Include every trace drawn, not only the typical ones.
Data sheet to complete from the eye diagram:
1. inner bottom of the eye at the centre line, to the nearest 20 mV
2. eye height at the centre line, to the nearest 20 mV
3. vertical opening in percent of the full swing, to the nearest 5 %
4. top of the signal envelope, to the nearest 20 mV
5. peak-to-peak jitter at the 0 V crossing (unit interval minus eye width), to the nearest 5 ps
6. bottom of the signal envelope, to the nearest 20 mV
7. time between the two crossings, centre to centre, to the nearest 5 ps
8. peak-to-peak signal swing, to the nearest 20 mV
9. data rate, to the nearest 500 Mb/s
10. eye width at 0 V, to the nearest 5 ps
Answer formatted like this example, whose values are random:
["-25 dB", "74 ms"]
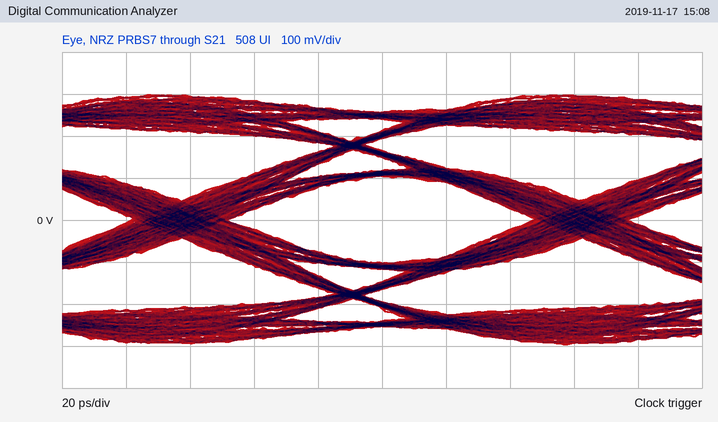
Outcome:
["-100 mV", "200 mV", "35 %", "300 mV", "30 ps", "-300 mV", "125 ps", "600 mV", "8.0 Gb/s", "95 ps"]
